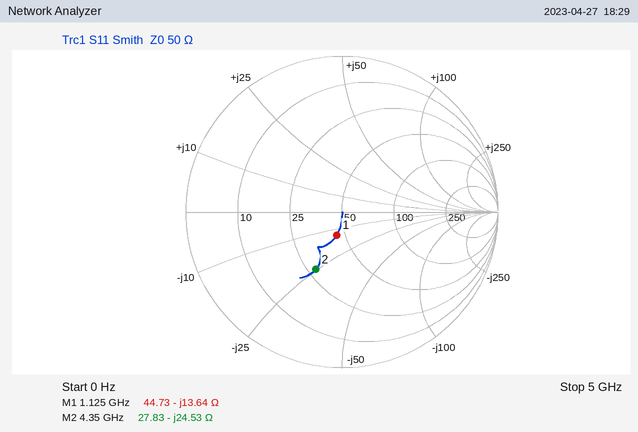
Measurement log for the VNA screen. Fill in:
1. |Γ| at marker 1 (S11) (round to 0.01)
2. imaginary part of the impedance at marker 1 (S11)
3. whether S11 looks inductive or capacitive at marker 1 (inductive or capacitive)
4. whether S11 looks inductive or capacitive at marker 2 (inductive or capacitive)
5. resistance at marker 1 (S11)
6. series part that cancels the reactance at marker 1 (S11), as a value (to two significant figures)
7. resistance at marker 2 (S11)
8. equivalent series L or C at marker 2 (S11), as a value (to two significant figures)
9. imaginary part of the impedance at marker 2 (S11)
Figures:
0.15
-13.64 Ω
capacitive
capacitive
44.73 Ω
1.9 nH
27.83 Ω
1.5 pF
-24.53 Ω
